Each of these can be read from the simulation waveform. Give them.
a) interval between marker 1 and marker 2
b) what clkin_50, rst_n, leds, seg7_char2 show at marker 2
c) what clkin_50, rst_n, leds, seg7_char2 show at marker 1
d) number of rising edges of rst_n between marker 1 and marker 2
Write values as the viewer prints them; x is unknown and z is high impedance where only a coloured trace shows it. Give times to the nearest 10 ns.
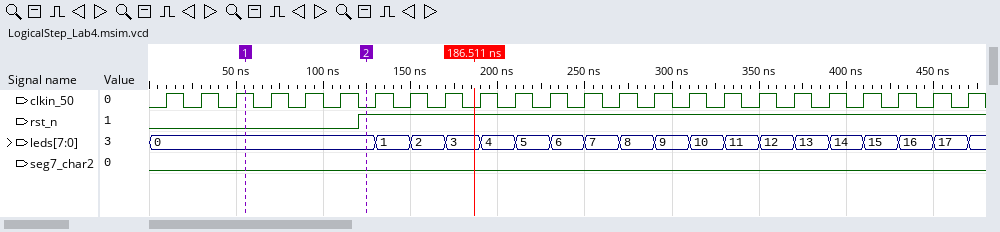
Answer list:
70 ns
clkin_50=0, rst_n=1, leds=0, seg7_char2=0
clkin_50=1, rst_n=0, leds=0, seg7_char2=0
1
